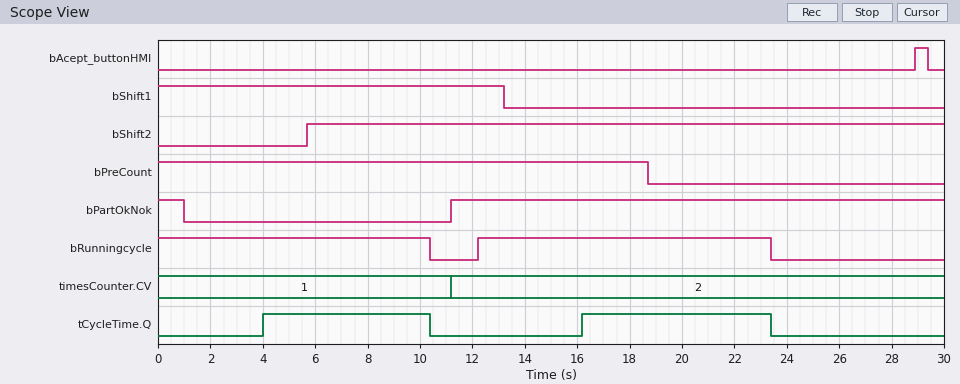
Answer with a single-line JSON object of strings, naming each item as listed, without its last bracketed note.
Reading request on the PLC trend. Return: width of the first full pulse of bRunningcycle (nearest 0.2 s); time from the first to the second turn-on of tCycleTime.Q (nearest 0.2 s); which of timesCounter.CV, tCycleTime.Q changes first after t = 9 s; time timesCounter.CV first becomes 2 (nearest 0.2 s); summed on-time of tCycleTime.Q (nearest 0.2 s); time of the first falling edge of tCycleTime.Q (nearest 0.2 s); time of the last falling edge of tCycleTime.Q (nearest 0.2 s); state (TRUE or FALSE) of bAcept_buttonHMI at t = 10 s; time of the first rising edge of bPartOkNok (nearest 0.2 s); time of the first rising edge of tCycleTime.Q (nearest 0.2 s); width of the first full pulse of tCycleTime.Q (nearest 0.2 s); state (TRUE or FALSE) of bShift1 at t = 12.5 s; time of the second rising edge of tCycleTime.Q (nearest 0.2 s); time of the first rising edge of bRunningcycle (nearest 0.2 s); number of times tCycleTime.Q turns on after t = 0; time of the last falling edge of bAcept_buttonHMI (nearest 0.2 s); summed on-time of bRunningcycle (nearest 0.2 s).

{"width of the first full pulse of bRunningcycle": "11.2 s", "time from the first to the second turn-on of tCycleTime.Q": "12.2 s", "which of timesCounter.CV, tCycleTime.Q changes first after t = 9 s": "tCycleTime.Q", "time timesCounter.CV first becomes 2": "11.2 s", "summed on-time of tCycleTime.Q": "13.6 s", "time of the first falling edge of tCycleTime.Q": "10.4 s", "time of the last falling edge of tCycleTime.Q": "23.4 s", "state (TRUE or FALSE) of bAcept_buttonHMI at t = 10 s": "FALSE", "time of the first rising edge of bPartOkNok": "11.2 s", "time of the first rising edge of tCycleTime.Q": "4.0 s", "width of the first full pulse of tCycleTime.Q": "6.4 s", "state (TRUE or FALSE) of bShift1 at t = 12.5 s": "TRUE", "time of the second rising edge of tCycleTime.Q": "16.2 s", "time of the first rising edge of bRunningcycle": "12.2 s", "number of times tCycleTime.Q turns on after t = 0": "2", "time of the last falling edge of bAcept_buttonHMI": "29.4 s", "summed on-time of bRunningcycle": "21.6 s"}
